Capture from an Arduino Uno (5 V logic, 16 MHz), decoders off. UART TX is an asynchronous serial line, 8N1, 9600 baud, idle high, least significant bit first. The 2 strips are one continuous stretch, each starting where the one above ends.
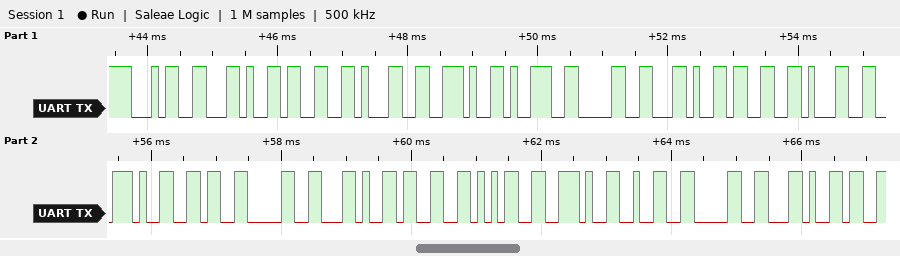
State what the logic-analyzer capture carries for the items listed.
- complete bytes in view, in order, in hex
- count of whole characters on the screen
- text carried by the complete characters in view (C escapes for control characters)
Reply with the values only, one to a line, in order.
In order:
0x34 0x2C 0x33 0x31 0x2E 0x39 0x30 0x2C 0x33 0x31 0x2E 0x36 0x30 0x2C 0x33 0x35 0x2E 0x32 0x30 0x2C
20
"4,31.90,31.60,35.20,"
